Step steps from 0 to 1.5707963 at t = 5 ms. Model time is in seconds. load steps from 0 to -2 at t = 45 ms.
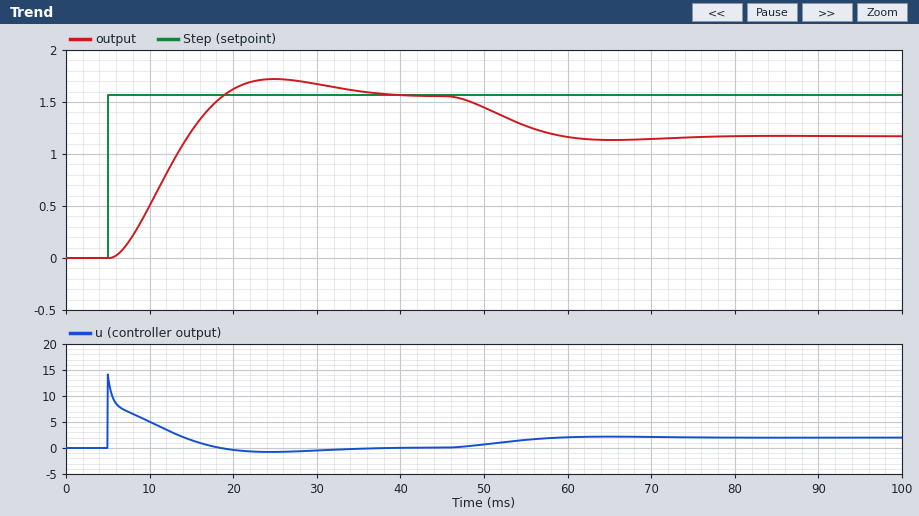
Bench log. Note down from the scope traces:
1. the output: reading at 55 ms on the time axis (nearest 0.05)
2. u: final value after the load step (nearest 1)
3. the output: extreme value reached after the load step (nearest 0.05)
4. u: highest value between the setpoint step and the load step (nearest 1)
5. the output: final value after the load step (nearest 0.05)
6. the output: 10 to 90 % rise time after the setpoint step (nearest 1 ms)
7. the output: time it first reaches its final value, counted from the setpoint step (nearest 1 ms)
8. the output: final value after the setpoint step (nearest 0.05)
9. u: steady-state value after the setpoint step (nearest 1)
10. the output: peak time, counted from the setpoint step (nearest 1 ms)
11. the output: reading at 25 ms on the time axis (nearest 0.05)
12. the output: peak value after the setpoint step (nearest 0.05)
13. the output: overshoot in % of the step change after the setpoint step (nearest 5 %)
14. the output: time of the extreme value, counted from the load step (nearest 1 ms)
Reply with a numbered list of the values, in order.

1. 1.25
2. 2
3. 1.15
4. 14
5. 1.15
6. 9 ms
7. 14 ms
8. 1.55
9. 0
10. 20 ms
11. 1.70
12. 1.70
13. 10 %
14. 20 ms
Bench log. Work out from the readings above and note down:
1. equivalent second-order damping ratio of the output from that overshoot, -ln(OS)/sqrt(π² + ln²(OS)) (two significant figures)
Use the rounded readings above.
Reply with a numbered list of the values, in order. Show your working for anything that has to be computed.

1. ln(0.1) = -2.303; 2.303 / sqrt(9.870 + 5.302) = 0.59
